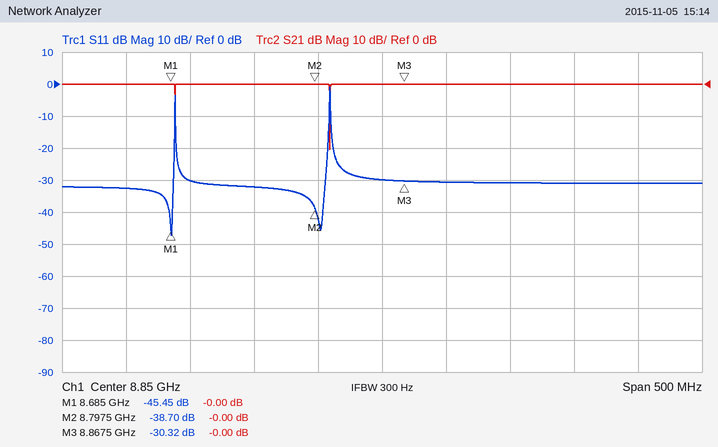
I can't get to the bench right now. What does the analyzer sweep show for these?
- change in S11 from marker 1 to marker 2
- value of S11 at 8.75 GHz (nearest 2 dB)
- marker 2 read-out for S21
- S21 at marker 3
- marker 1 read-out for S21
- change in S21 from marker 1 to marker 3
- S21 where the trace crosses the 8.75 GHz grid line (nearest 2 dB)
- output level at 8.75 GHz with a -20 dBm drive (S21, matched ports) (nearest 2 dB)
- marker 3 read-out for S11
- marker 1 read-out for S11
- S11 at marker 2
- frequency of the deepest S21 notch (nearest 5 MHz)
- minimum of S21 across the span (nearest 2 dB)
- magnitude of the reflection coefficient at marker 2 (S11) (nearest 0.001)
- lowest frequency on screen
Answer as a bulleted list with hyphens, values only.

- 6.75 dB
- -32 dB
- -0.00 dB
- -0.00 dB
- -0.00 dB
- 0.00 dB
- 0 dB
- -20 dBm
- -30.32 dB
- -45.45 dB
- -38.70 dB
- 8.810 GHz
- -20 dB
- 0.012
- 8.6 GHz
